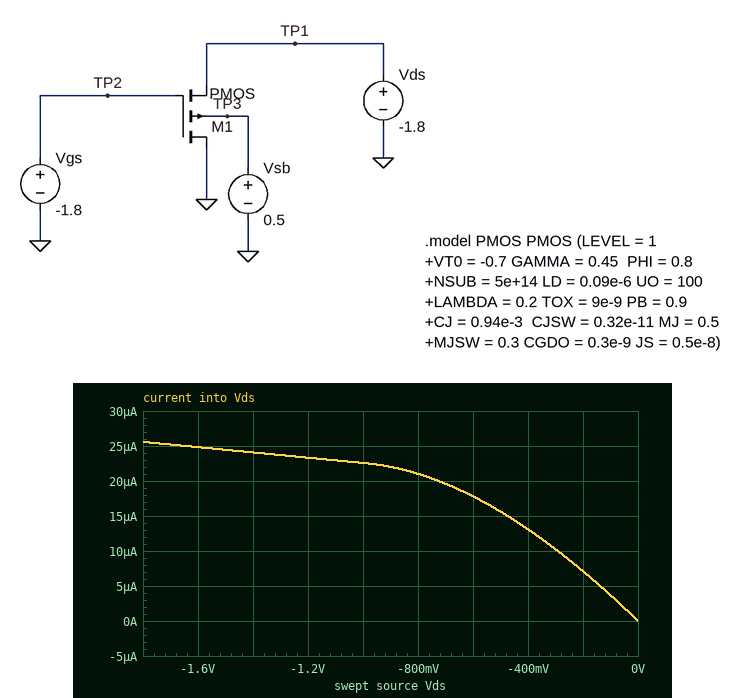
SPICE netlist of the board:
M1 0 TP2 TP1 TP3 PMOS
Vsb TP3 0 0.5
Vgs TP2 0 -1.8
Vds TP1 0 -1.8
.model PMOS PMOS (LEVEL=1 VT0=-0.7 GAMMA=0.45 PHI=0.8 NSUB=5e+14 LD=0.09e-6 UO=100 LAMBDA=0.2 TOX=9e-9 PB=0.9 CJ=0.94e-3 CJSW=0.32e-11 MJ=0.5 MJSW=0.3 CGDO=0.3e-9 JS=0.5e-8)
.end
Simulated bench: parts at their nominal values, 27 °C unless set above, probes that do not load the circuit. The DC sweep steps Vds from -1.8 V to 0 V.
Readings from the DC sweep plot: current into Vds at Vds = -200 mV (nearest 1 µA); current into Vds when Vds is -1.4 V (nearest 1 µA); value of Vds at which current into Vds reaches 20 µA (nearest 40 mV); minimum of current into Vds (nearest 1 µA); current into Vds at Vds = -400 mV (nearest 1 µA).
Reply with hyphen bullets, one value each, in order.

- 7 µA
- 24 µA
- -720 mV
- 0 A
- 13 µA
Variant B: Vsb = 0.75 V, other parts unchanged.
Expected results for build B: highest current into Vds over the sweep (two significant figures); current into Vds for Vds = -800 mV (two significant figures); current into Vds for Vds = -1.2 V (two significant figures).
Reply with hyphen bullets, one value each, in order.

- 23 µA
- 19 µA
- 21 µA
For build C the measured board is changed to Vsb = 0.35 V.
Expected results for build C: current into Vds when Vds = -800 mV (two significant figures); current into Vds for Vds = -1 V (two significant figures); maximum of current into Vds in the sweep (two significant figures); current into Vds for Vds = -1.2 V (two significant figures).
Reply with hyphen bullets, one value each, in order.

- 22 µA
- 24 µA
- 27 µA
- 25 µA
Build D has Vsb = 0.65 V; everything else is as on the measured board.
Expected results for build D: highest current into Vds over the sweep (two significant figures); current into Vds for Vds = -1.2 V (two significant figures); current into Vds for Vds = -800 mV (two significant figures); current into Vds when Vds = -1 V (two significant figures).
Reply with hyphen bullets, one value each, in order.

- 24 µA
- 22 µA
- 20 µA
- 21 µA
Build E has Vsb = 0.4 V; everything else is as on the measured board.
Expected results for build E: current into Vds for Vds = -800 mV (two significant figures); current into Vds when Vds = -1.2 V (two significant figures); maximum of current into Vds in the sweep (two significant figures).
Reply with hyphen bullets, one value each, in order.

- 22 µA
- 24 µA
- 27 µA
